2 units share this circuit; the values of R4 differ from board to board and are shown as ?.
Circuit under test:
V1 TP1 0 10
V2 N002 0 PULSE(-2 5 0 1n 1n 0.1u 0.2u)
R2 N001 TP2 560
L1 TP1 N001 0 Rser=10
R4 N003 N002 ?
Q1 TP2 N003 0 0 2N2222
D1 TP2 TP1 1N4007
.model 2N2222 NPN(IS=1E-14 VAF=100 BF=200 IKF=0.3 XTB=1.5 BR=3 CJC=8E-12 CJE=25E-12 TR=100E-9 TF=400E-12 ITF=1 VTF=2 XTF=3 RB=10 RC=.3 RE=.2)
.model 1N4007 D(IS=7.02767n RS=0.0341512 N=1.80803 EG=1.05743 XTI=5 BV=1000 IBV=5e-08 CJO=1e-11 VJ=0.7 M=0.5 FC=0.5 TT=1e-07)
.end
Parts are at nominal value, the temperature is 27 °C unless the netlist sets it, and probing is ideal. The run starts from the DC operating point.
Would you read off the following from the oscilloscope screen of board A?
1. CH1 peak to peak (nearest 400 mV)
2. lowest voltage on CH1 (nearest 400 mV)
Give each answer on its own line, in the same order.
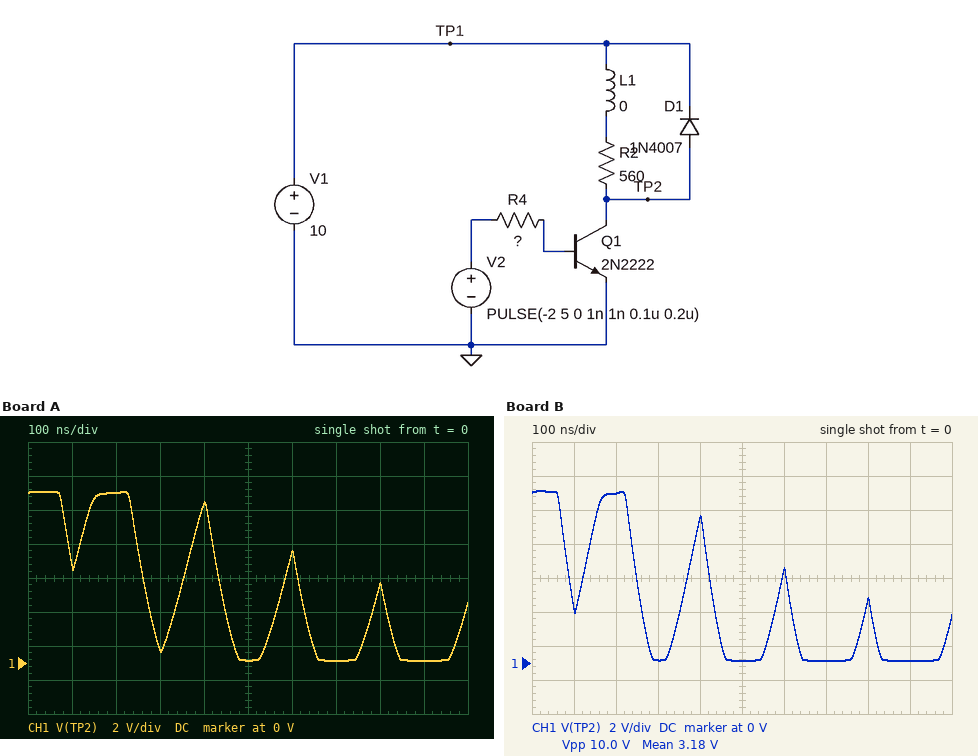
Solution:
10.0 V
0 V
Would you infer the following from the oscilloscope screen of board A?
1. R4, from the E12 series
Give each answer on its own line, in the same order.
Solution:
5.6 kΩ
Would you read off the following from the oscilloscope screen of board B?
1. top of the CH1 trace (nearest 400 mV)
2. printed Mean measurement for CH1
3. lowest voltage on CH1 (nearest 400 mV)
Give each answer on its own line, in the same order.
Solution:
10.0 V
3.18 V
0 V
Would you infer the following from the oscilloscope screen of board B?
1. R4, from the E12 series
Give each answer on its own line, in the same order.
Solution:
4.7 kΩ
